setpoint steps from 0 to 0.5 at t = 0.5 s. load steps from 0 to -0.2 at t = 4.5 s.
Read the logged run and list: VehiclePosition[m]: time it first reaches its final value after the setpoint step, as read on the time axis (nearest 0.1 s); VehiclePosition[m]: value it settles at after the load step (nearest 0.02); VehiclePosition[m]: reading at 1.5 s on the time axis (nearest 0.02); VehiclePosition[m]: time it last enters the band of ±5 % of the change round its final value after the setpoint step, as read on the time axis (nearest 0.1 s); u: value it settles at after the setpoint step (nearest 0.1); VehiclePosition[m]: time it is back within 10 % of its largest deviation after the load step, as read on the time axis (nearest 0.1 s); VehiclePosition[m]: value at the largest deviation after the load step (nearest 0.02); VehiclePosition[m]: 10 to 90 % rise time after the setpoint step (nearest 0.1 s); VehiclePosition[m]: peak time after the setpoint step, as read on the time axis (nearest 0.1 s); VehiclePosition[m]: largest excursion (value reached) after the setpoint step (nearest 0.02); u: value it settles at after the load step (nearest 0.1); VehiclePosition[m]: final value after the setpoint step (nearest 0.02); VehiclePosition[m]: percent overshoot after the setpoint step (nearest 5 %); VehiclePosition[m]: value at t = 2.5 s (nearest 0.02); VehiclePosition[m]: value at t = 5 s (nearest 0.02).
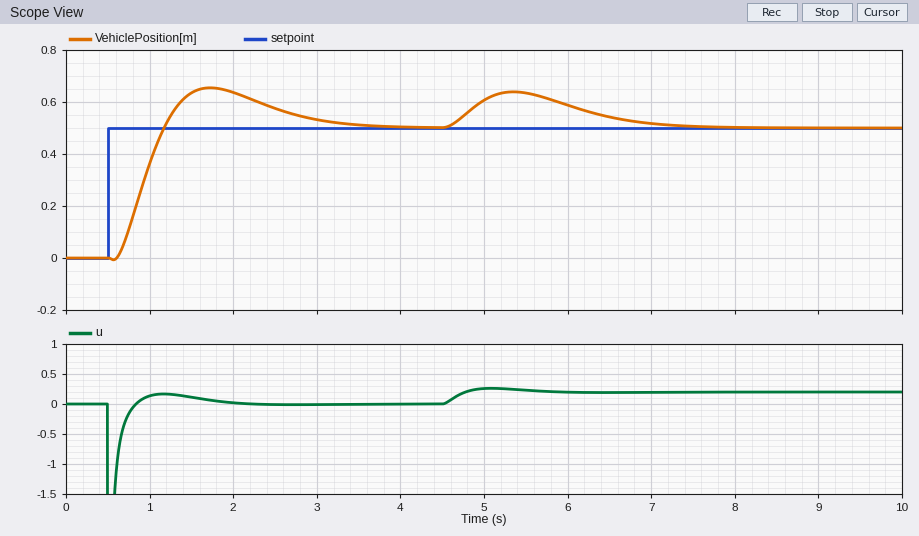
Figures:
1.2 s
0.50
0.64
3.1 s
0.0
7.1 s
0.64
0.4 s
1.7 s
0.66
0.2
0.50
30 %
0.58
0.60
